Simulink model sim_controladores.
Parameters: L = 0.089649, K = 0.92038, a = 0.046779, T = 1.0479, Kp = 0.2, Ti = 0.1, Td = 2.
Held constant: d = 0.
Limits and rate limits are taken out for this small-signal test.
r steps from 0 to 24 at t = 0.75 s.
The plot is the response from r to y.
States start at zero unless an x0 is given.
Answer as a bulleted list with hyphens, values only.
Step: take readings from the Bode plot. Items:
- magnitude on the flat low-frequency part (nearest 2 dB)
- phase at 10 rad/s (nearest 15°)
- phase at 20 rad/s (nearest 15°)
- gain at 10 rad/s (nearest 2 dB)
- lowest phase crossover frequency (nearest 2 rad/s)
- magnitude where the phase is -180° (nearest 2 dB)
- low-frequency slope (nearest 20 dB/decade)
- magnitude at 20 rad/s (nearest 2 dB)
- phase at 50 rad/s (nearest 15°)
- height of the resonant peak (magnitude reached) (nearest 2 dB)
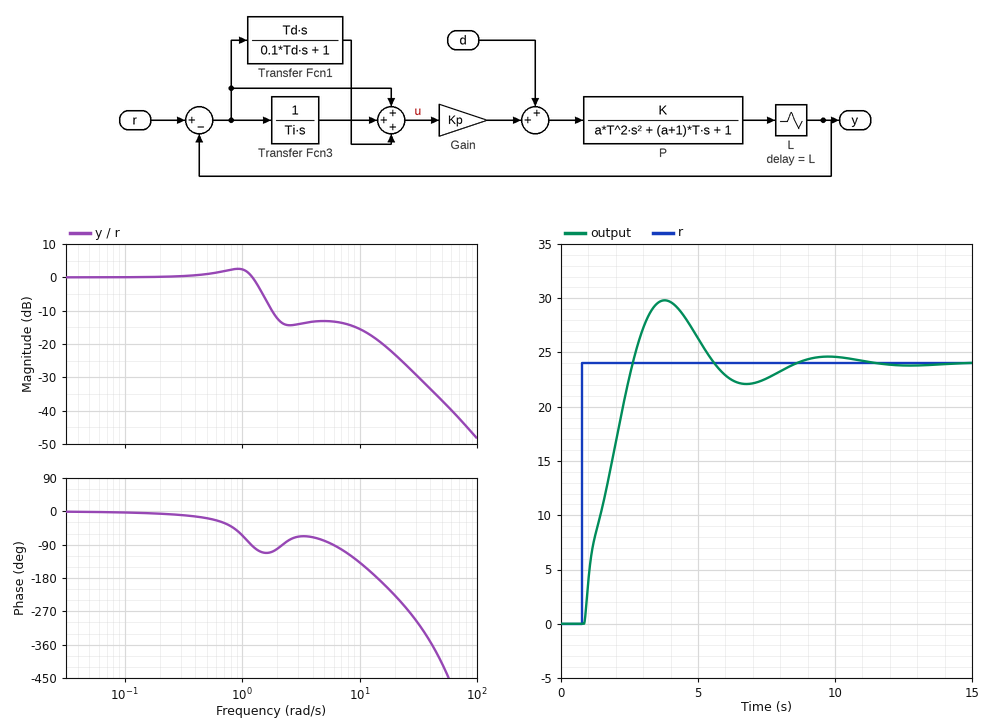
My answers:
- 0 dB
- -135°
- -225°
- -16 dB
- 14 rad/s
- -18 dB
- 0 dB/decade
- -24 dB
- -405°
- 2 dB
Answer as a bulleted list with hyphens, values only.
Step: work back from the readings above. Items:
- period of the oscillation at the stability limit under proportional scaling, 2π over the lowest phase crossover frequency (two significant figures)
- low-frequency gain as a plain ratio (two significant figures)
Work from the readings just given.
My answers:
- 0.45 s
- 1.0
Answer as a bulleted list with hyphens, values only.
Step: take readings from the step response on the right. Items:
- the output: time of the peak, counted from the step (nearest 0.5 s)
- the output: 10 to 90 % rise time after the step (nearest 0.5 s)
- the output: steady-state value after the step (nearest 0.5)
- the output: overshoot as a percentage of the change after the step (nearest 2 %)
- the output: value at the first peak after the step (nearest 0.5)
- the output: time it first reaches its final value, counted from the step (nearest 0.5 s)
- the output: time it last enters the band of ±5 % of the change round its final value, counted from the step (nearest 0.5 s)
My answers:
- 3.0 s
- 1.5 s
- 24.0
- 24 %
- 30.0
- 2.0 s
- 7.0 s
